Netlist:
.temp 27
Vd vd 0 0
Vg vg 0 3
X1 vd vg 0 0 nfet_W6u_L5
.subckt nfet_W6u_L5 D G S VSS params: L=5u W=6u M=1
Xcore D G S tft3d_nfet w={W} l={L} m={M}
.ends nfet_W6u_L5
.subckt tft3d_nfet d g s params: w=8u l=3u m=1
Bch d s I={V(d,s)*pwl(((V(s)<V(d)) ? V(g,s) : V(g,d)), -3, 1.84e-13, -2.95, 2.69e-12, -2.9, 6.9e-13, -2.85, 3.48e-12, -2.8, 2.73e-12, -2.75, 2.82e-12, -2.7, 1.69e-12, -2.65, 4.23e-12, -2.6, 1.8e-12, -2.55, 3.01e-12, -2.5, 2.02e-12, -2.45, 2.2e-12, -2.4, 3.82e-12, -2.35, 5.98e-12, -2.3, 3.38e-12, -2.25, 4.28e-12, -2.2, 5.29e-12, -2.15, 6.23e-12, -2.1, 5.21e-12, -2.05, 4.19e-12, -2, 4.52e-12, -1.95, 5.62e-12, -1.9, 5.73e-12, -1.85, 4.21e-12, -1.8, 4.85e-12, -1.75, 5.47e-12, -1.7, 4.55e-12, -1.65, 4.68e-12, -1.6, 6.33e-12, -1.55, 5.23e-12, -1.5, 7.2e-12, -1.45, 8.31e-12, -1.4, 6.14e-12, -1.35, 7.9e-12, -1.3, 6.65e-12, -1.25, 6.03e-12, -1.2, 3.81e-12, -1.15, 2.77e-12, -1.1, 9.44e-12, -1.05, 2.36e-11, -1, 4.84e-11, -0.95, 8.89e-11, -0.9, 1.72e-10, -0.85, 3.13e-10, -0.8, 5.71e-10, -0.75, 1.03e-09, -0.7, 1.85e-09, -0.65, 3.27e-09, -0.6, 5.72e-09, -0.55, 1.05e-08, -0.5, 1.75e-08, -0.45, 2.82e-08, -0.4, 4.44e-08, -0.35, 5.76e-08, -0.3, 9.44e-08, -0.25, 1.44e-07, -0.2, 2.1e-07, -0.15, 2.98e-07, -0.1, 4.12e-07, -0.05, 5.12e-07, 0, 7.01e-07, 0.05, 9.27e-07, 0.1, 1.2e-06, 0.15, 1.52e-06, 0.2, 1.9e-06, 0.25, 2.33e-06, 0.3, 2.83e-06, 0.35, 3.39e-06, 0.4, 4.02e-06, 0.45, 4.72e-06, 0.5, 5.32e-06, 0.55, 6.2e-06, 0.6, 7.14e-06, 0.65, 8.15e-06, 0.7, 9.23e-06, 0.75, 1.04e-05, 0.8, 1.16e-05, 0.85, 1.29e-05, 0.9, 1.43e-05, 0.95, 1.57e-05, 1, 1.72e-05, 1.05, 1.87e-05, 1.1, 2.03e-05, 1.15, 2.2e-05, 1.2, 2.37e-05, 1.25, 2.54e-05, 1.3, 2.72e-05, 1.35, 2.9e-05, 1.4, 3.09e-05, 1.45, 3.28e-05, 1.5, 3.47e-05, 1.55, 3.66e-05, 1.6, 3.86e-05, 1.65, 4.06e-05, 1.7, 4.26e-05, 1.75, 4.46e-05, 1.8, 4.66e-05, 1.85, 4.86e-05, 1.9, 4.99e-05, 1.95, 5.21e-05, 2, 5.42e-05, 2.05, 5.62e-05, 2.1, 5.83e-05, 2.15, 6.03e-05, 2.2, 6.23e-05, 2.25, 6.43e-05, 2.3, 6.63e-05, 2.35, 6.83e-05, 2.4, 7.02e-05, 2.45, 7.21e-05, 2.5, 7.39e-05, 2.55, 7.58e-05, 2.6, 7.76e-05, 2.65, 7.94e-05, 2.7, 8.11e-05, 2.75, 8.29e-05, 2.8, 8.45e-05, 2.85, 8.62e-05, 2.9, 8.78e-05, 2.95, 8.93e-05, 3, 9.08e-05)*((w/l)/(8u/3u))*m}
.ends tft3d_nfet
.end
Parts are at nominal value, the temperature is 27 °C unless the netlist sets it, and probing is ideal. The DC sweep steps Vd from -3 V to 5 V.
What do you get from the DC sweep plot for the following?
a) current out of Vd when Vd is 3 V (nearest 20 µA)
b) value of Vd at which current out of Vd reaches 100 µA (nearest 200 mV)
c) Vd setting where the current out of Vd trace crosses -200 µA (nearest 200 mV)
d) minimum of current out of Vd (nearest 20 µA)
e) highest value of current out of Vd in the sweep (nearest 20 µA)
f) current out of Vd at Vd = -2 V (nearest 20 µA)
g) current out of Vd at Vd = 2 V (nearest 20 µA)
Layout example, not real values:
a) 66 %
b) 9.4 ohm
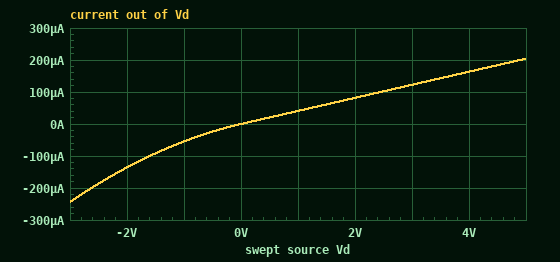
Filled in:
a) 120 µA
b) 2.4 V
c) -2.6 V
d) -240 µA
e) 200 µA
f) -140 µA
g) 80 µA
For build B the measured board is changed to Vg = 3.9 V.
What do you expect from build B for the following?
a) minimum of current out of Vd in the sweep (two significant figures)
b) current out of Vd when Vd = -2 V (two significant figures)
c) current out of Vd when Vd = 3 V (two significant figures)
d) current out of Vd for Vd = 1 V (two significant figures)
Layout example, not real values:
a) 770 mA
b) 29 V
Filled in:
a) -280 µA
b) -160 µA
c) 160 µA
d) 53 µA
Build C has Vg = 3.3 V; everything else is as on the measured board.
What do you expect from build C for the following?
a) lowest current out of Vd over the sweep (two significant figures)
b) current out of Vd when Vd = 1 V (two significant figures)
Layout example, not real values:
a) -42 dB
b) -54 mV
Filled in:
a) -260 µA
b) 45 µA
